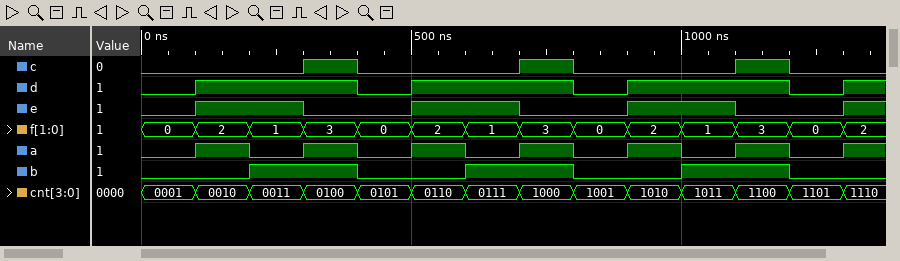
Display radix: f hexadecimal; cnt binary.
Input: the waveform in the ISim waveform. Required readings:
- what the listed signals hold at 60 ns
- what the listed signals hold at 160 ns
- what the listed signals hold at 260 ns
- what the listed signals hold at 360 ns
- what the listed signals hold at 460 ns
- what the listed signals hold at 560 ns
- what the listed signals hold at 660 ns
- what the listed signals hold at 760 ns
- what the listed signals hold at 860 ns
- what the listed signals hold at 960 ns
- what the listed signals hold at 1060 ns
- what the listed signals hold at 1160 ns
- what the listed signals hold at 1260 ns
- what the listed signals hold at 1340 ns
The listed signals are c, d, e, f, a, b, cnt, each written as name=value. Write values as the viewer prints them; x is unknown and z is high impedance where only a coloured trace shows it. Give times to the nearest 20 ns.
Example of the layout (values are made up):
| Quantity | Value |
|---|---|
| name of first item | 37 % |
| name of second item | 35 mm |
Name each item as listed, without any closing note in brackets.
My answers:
| Quantity | Value |
|---|---|
| what the listed signals hold at 60 ns | c=0, d=0, e=0, f=0, a=0, b=0, cnt=0001 |
| what the listed signals hold at 160 ns | c=0, d=1, e=1, f=2, a=1, b=0, cnt=0010 |
| what the listed signals hold at 260 ns | c=0, d=1, e=1, f=1, a=0, b=1, cnt=0011 |
| what the listed signals hold at 360 ns | c=1, d=1, e=0, f=3, a=1, b=1, cnt=0100 |
| what the listed signals hold at 460 ns | c=0, d=0, e=0, f=0, a=0, b=0, cnt=0101 |
| what the listed signals hold at 560 ns | c=0, d=1, e=1, f=2, a=1, b=0, cnt=0110 |
| what the listed signals hold at 660 ns | c=0, d=1, e=1, f=1, a=0, b=1, cnt=0111 |
| what the listed signals hold at 760 ns | c=1, d=1, e=0, f=3, a=1, b=1, cnt=1000 |
| what the listed signals hold at 860 ns | c=0, d=0, e=0, f=0, a=0, b=0, cnt=1001 |
| what the listed signals hold at 960 ns | c=0, d=1, e=1, f=2, a=1, b=0, cnt=1010 |
| what the listed signals hold at 1060 ns | c=0, d=1, e=1, f=1, a=0, b=1, cnt=1011 |
| what the listed signals hold at 1160 ns | c=1, d=1, e=0, f=3, a=1, b=1, cnt=1100 |
| what the listed signals hold at 1260 ns | c=0, d=0, e=0, f=0, a=0, b=0, cnt=1101 |
| what the listed signals hold at 1340 ns | c=0, d=1, e=1, f=2, a=1, b=0, cnt=1110 |
